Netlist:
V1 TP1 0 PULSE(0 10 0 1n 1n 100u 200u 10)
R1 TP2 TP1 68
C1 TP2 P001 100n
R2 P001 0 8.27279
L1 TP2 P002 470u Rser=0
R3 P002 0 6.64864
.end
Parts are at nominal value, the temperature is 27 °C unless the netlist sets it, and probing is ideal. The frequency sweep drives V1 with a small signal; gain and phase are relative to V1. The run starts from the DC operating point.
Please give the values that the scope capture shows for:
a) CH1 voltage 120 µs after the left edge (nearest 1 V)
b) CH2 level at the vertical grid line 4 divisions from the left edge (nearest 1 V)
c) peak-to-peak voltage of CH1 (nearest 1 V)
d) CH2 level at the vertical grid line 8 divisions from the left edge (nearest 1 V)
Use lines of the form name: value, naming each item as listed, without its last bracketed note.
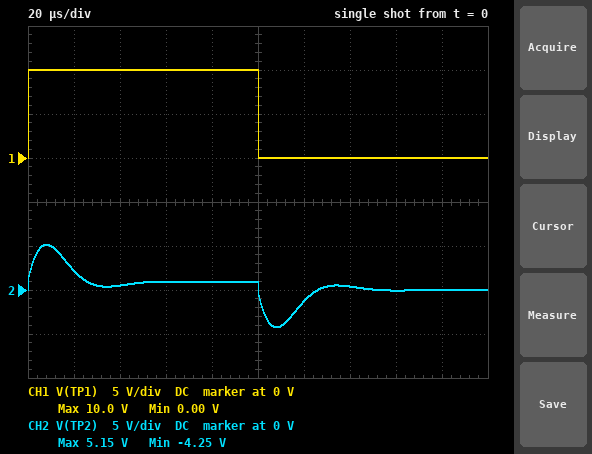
CH1 voltage 120 µs after the left edge: 0 V
CH2 level at the vertical grid line 4 divisions from the left edge: 1 V
peak-to-peak voltage of CH1: 10 V
CH2 level at the vertical grid line 8 divisions from the left edge: 0 V
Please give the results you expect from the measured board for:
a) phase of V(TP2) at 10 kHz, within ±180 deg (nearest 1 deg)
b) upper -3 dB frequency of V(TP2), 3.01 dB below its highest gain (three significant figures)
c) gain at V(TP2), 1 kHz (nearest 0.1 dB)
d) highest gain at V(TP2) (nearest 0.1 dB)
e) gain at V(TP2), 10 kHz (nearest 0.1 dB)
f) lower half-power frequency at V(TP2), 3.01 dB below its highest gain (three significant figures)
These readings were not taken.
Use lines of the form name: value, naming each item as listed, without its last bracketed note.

phase of V(TP2) at 10 kHz, within ±180 deg: 49 deg
upper -3 dB frequency of V(TP2), 3.01 dB below its highest gain: 39.5 kHz
gain at V(TP2), 1 kHz: -20.2 dB
highest gain at V(TP2): -1.7 dB
gain at V(TP2), 10 kHz: -7.3 dB
lower half-power frequency at V(TP2), 3.01 dB below its highest gain: 13.4 kHz
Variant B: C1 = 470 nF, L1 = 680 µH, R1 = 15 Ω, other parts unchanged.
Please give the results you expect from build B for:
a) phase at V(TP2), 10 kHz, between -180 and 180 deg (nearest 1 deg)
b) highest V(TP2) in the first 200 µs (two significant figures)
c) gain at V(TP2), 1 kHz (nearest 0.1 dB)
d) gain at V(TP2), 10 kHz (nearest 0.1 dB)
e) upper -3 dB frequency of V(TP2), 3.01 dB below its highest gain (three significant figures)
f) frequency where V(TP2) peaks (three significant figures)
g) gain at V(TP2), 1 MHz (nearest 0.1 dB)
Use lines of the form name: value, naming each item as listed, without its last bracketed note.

phase at V(TP2), 10 kHz, between -180 and 180 deg: -4 deg
highest V(TP2) in the first 200 µs: 7.2 V
gain at V(TP2), 1 kHz: -8.9 dB
gain at V(TP2), 10 kHz: -1.3 dB
upper -3 dB frequency of V(TP2), 3.01 dB below its highest gain: 24.5 kHz
frequency where V(TP2) peaks: 8.69 kHz
gain at V(TP2), 1 MHz: -9.0 dB
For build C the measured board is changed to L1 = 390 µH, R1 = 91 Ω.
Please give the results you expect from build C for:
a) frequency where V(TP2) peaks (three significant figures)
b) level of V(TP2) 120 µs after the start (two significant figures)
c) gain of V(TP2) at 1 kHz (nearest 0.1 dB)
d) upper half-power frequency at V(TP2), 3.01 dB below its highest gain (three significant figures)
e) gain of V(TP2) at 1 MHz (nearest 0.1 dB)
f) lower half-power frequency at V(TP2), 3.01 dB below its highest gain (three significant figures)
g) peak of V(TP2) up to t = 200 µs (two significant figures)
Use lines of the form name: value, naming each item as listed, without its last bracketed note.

frequency where V(TP2) peaks: 25.3 kHz
level of V(TP2) 120 µs after the start: -410 mV
gain of V(TP2) at 1 kHz: -22.8 dB
upper half-power frequency at V(TP2), 3.01 dB below its highest gain: 38.7 kHz
gain of V(TP2) at 1 MHz: -21.4 dB
lower half-power frequency at V(TP2), 3.01 dB below its highest gain: 16.6 kHz
peak of V(TP2) up to t = 200 µs: 4.1 V
